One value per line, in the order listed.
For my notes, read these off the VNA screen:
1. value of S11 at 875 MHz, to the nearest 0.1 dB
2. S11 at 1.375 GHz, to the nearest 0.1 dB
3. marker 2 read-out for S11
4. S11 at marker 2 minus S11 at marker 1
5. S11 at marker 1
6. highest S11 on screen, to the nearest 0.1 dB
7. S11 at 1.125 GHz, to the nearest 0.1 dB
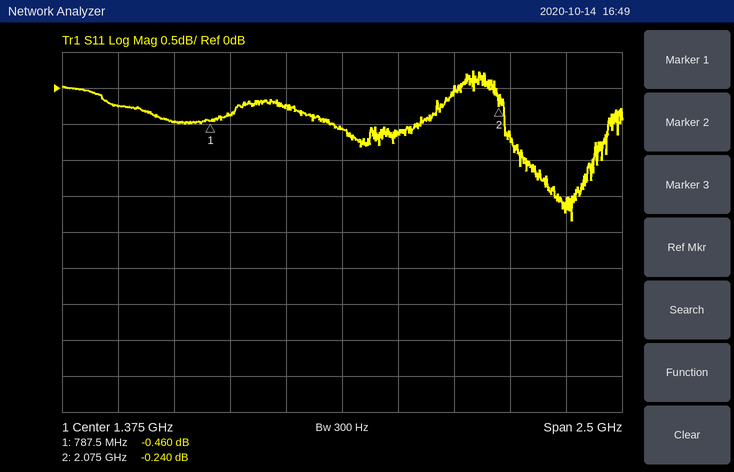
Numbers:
-0.4 dB
-0.6 dB
-0.240 dB
0.220 dB
-0.460 dB
0.2 dB
-0.2 dB
